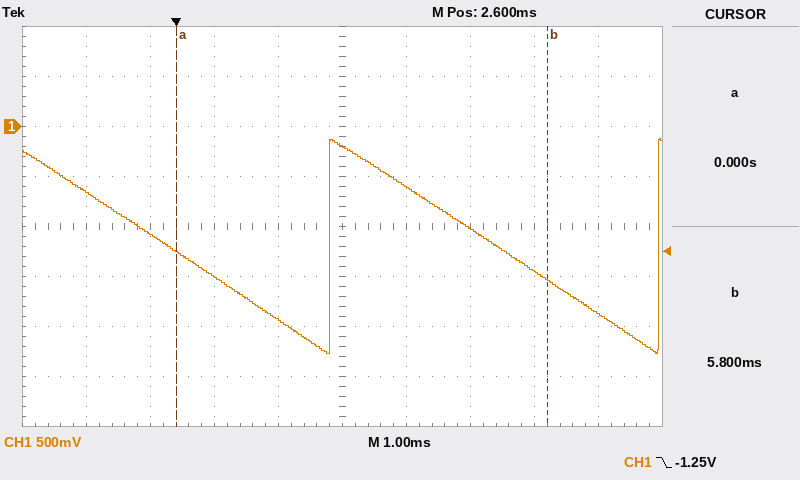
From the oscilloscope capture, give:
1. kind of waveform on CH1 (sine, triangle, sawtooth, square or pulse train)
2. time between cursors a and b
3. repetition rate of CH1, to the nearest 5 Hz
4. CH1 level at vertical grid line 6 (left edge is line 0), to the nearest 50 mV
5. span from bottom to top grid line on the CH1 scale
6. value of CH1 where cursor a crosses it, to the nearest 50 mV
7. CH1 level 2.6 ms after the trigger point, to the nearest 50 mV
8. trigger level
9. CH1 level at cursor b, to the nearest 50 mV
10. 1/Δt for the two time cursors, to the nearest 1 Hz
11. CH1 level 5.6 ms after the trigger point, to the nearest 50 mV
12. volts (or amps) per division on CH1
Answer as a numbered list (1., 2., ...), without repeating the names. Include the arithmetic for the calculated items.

1. sawtooth
2. 5.8 ms − (0 s) = 5.8 ms
3. 195 Hz
4. -600 mV
5. 4 V
6. -1.25 V
7. -200 mV
8. -1.25 V
9. -1.55 V
10. 1 / 5.8 ms ≈ 172 Hz
11. -1.45 V
12. 500 mV
